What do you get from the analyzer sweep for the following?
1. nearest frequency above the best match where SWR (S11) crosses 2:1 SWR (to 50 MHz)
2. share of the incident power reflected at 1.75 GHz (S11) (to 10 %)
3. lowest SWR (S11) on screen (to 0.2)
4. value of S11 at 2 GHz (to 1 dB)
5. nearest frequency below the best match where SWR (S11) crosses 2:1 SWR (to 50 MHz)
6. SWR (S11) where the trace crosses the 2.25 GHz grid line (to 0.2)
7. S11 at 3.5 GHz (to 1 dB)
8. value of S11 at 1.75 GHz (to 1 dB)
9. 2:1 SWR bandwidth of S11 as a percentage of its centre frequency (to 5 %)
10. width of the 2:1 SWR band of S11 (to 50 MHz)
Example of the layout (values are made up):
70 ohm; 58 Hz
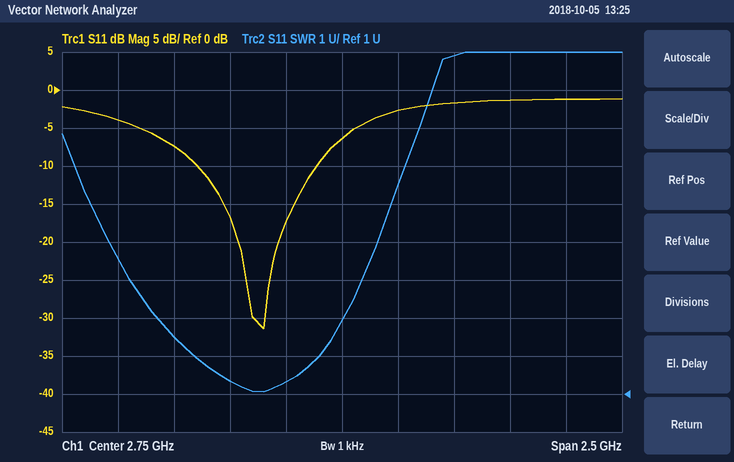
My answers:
2.65 GHz; 40 %; 1.0; -7 dB; 2.10 GHz; 1.4; -1 dB; -4 dB; 25 %; 550 MHz
